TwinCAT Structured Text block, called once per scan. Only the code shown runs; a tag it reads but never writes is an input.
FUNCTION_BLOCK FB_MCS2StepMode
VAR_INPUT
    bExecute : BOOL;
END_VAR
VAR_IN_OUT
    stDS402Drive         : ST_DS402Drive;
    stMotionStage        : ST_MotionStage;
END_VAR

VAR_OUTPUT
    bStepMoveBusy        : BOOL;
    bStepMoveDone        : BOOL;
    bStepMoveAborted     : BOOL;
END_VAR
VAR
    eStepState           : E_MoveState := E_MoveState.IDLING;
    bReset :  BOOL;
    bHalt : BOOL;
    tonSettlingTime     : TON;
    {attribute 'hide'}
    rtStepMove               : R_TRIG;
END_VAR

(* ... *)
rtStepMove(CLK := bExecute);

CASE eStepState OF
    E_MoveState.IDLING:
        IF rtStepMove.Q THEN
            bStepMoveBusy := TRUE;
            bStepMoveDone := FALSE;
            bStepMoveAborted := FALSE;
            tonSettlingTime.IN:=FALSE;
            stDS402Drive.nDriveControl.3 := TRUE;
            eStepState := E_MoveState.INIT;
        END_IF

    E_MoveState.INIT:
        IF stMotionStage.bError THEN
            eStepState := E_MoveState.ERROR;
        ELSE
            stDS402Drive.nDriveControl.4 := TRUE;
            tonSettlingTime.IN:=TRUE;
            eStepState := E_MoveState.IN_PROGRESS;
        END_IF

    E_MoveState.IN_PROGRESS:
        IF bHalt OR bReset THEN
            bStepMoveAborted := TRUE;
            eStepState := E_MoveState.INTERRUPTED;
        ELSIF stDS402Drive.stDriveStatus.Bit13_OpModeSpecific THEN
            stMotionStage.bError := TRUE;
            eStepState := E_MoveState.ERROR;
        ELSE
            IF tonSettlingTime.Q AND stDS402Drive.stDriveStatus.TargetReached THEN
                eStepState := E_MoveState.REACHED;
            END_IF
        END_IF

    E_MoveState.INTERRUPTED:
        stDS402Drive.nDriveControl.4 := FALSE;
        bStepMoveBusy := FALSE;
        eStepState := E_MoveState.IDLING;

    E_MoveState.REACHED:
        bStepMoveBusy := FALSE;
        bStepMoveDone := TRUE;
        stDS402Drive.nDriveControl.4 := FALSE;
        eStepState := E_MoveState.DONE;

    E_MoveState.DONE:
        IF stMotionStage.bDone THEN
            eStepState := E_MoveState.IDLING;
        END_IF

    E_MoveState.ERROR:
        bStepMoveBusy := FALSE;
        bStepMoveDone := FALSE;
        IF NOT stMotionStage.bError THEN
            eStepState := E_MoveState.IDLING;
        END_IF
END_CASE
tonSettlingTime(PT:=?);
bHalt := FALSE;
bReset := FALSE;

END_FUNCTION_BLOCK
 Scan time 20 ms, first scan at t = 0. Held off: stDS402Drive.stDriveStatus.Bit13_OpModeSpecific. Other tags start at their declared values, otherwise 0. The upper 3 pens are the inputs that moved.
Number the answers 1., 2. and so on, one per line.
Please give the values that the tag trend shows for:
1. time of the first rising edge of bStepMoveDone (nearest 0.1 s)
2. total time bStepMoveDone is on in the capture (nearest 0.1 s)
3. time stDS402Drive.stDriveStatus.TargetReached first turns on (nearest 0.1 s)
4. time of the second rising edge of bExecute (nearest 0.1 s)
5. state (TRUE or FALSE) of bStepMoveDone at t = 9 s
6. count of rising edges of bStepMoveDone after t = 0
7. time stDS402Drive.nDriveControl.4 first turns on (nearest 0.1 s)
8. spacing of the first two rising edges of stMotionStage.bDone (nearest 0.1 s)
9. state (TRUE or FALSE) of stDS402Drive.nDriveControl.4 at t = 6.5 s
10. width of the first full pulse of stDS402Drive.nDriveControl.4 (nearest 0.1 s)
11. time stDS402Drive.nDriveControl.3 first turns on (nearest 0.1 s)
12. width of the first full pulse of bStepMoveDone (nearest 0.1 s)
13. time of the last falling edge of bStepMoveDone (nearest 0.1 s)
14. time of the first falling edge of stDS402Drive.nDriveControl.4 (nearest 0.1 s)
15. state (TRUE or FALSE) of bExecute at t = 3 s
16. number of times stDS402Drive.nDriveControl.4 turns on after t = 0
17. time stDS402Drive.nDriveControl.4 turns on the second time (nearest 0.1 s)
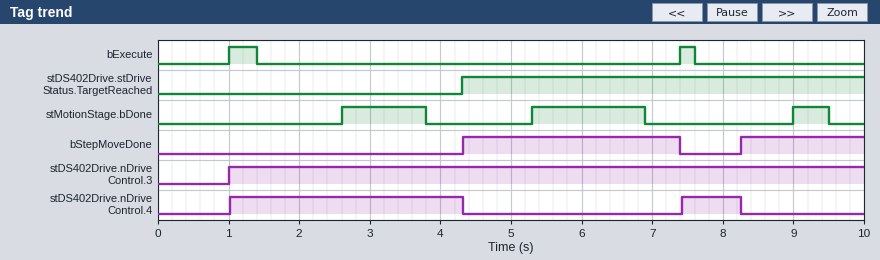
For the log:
1. 4.3 s
2. 4.8 s
3. 4.3 s
4. 7.4 s
5. TRUE
6. 2
7. 1.0 s
8. 2.7 s
9. FALSE
10. 3.3 s
11. 1.0 s
12. 3.1 s
13. 7.4 s
14. 4.3 s
15. FALSE
16. 2
17. 7.4 s
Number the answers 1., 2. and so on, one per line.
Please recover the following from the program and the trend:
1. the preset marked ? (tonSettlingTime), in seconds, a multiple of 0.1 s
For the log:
1. 0.8 s
